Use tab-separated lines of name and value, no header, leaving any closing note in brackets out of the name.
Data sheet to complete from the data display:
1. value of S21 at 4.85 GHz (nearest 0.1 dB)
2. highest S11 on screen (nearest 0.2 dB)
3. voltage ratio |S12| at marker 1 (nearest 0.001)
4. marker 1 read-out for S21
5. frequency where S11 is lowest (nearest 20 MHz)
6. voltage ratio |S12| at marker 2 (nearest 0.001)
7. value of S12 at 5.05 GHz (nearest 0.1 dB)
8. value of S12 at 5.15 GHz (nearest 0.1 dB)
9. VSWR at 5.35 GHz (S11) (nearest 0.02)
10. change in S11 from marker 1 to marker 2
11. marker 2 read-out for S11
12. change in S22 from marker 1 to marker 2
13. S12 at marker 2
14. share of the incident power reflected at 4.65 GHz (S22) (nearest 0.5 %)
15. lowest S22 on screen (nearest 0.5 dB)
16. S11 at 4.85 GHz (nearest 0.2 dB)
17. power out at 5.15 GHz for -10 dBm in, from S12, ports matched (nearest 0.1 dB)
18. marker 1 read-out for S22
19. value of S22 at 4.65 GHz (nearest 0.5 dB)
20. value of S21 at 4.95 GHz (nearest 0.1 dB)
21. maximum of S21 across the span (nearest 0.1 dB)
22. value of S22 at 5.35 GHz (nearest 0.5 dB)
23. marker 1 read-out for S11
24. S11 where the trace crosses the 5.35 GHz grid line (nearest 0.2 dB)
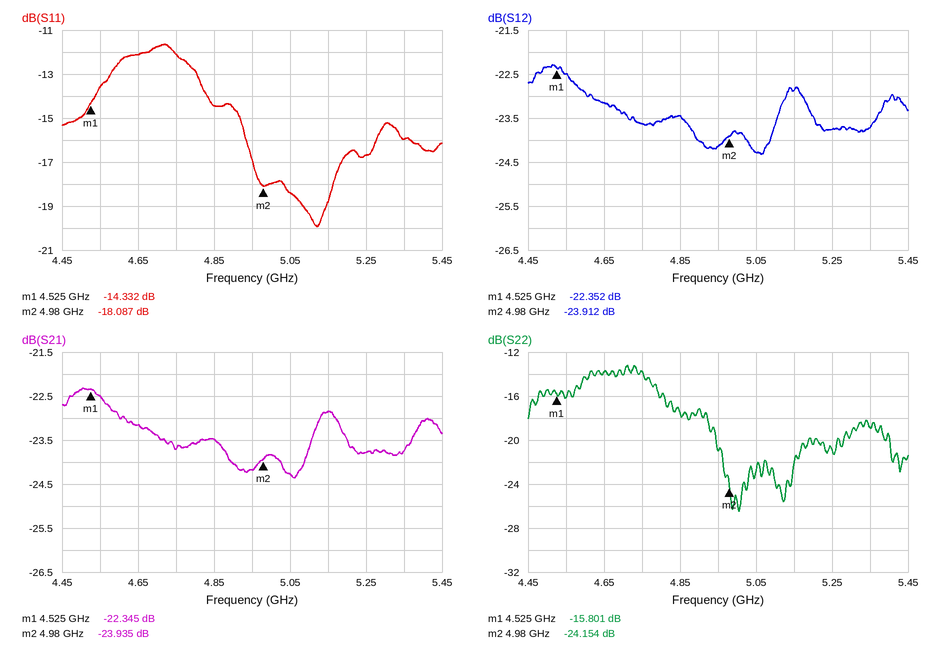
value of S21 at 4.85 GHz	-23.5 dB
highest S11 on screen	-11.6 dB
voltage ratio |S12| at marker 1	0.076
marker 1 read-out for S21	-22.345 dB
frequency where S11 is lowest	5.12 GHz
voltage ratio |S12| at marker 2	0.064
value of S12 at 5.05 GHz	-24.3 dB
value of S12 at 5.15 GHz	-22.9 dB
VSWR at 5.35 GHz (S11)	1.38
change in S11 from marker 1 to marker 2	-3.755 dB
marker 2 read-out for S11	-18.087 dB
change in S22 from marker 1 to marker 2	-8.353 dB
S12 at marker 2	-23.912 dB
share of the incident power reflected at 4.65 GHz (S22)	4.0 %
lowest S22 on screen	-26.5 dB
S11 at 4.85 GHz	-14.4 dB
power out at 5.15 GHz for -10 dBm in, from S12, ports matched	-32.9 dBm
marker 1 read-out for S22	-15.801 dB
value of S22 at 4.65 GHz	-14.0 dB
value of S21 at 4.95 GHz	-24.2 dB
maximum of S21 across the span	-22.3 dB
value of S22 at 5.35 GHz	-19.0 dB
marker 1 read-out for S11	-14.332 dB
S11 where the trace crosses the 5.35 GHz grid line	-16.0 dB
